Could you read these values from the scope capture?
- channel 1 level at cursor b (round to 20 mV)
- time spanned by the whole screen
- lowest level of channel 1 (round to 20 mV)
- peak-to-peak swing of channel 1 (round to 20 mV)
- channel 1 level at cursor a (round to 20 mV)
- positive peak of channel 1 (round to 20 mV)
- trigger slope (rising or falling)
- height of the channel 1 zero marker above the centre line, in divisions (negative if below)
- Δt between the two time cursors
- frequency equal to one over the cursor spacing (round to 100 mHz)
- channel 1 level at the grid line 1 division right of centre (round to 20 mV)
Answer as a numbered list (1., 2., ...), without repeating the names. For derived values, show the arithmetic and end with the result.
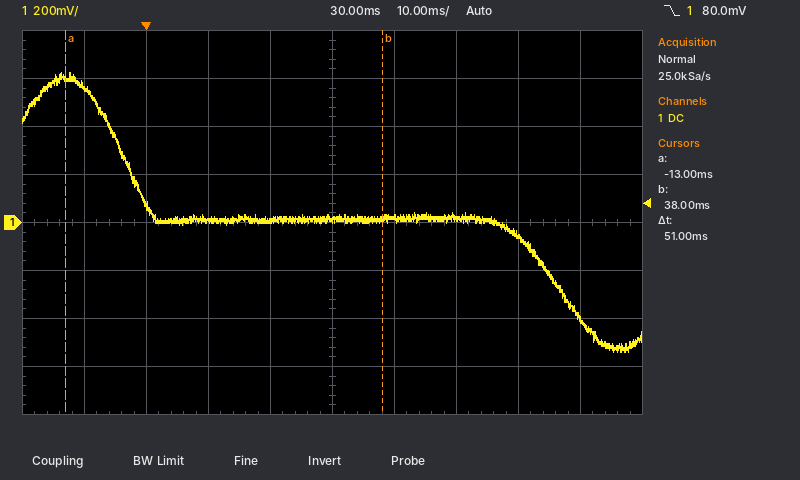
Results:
1. 20 mV
2. 100 ms
3. -540 mV
4. 620 mV − (-540 mV) = 1.16 V
5. 600 mV
6. 620 mV
7. falling
8. 0.0 div
9. 51 ms
10. 1 / 51 ms ≈ 19.6 Hz
11. 20 mV
